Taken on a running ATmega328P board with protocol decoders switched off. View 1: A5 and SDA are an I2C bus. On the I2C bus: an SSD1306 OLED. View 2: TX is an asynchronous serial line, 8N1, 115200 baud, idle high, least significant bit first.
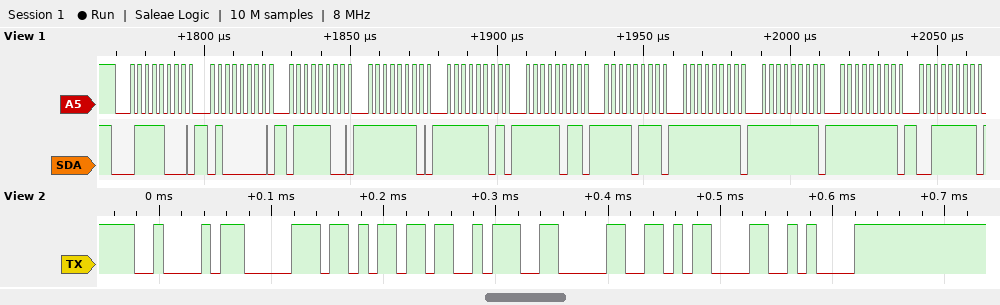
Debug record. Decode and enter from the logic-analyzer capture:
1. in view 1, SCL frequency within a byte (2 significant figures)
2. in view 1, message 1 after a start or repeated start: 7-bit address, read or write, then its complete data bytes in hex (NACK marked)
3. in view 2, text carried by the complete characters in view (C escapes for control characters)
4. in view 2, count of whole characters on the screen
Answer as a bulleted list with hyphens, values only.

- 400 kHz
- 0x3C write: 40 7C FE FD FB F7 FF FF FF 3F
- "Bpm:0\r\n"
- 7
